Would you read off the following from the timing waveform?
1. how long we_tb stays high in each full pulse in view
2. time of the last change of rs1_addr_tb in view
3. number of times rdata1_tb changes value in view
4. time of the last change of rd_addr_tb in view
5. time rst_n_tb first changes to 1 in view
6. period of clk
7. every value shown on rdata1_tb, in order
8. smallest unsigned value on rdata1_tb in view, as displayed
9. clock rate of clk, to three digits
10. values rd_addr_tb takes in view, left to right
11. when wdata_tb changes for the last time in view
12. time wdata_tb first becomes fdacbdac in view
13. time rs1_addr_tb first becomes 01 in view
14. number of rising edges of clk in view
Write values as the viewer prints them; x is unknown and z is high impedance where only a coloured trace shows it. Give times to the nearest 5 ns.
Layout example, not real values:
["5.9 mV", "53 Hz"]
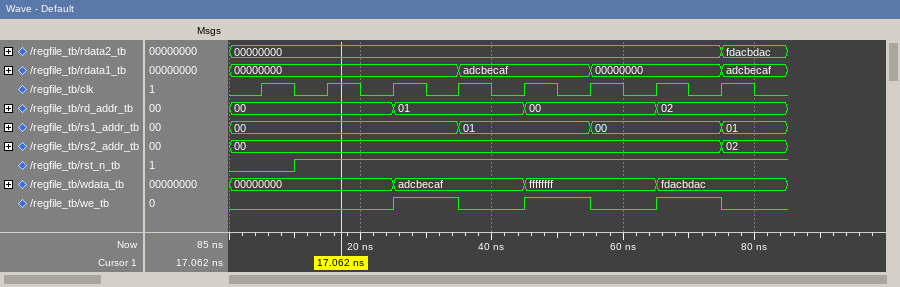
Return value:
["10 ns, 10 ns, 10 ns", "75 ns", "3", "65 ns", "10 ns", "10 ns", "00000000, adcbecaf, 00000000, adcbecaf", "00000000", "100 MHz", "00, 01, 00, 02", "65 ns", "65 ns", "35 ns", "8"]
